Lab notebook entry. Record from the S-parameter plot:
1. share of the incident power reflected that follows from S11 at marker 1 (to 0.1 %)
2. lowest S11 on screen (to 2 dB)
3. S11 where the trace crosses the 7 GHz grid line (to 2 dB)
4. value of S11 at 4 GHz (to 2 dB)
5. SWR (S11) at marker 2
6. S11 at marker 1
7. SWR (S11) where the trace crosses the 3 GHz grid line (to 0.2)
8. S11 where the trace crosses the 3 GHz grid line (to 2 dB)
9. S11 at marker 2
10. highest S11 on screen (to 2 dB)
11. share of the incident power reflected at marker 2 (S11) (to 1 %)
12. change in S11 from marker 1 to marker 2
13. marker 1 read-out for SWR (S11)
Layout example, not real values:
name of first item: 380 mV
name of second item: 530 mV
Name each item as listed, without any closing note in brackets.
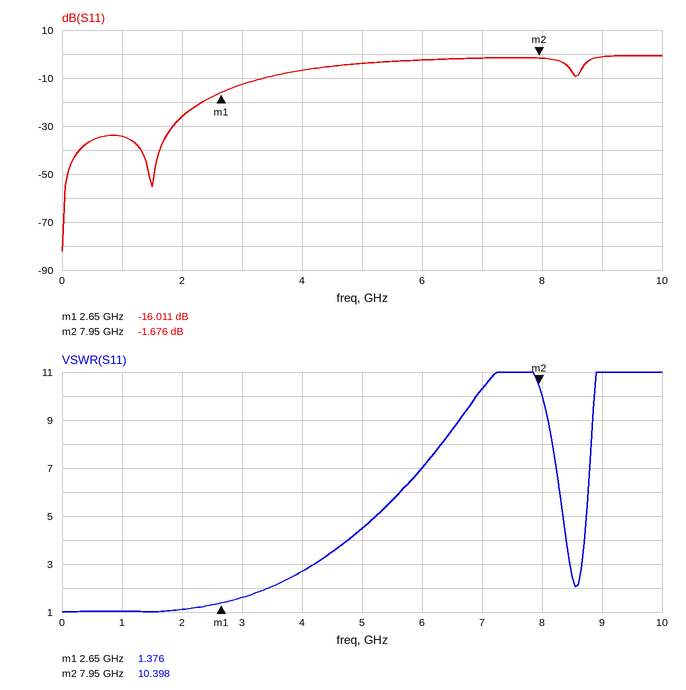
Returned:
share of the incident power reflected that follows from S11 at marker 1: 2.5 %
lowest S11 on screen: -82 dB
S11 where the trace crosses the 7 GHz grid line: -2 dB
value of S11 at 4 GHz: -6 dB
SWR (S11) at marker 2: 10.398
S11 at marker 1: -16.011 dB
SWR (S11) where the trace crosses the 3 GHz grid line: 1.6
S11 where the trace crosses the 3 GHz grid line: -12 dB
S11 at marker 2: -1.676 dB
highest S11 on screen: 0 dB
share of the incident power reflected at marker 2 (S11): 68 %
change in S11 from marker 1 to marker 2: 14.335 dB
marker 1 read-out for SWR: 1.376
